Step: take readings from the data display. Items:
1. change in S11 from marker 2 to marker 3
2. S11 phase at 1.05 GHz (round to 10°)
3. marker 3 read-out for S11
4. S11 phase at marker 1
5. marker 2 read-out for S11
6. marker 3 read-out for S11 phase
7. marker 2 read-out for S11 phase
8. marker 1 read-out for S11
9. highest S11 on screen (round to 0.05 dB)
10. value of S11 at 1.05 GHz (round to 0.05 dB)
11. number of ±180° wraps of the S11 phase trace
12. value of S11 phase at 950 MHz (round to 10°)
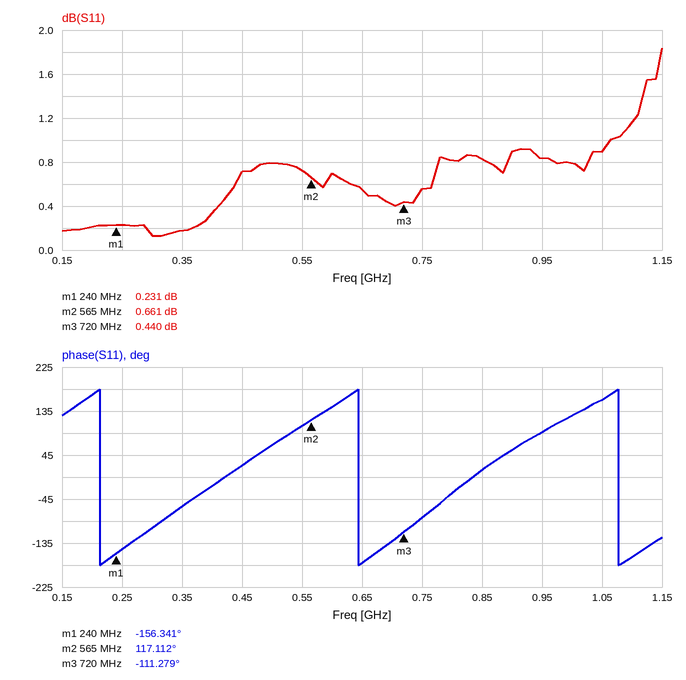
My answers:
-0.221 dB
160°
0.440 dB
-156.341°
0.661 dB
-111.279°
117.112°
0.231 dB
1.85 dB
0.90 dB
3
90°
